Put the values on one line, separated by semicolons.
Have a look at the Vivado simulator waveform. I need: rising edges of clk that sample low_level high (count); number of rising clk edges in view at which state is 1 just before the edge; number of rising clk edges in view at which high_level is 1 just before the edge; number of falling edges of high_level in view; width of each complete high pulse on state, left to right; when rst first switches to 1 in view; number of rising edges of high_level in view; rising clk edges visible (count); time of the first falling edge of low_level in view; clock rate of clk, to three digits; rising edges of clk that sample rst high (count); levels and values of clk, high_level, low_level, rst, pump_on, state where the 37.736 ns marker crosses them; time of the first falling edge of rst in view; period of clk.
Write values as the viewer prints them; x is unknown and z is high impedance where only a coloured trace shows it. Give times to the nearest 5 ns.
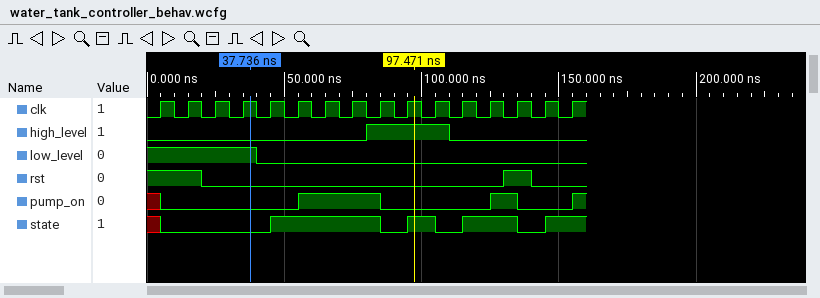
4; 8; 3; 1; 40 ns, 10 ns, 20 ns; 130 ns; 1; 16; 40 ns; 100 MHz; 3; clk=1, high_level=0, low_level=1, rst=0, pump_on=0, state=0; 20 ns; 10 ns
